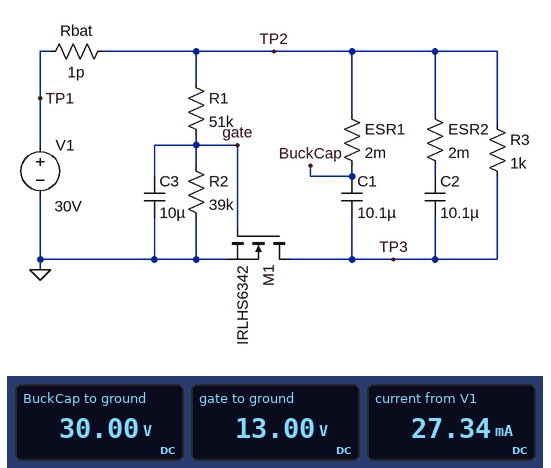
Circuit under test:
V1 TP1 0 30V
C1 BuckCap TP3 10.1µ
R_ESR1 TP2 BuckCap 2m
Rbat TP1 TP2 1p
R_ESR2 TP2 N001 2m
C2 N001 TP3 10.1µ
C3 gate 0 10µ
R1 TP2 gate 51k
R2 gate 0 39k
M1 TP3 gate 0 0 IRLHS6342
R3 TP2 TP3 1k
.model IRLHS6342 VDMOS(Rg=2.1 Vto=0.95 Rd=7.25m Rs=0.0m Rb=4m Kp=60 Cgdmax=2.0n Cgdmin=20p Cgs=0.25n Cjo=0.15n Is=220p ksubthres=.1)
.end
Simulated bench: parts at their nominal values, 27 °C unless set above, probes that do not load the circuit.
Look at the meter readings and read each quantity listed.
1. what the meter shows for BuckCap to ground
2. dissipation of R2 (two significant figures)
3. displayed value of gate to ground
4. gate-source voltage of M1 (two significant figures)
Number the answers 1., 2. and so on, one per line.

1. 30.00 V
2. 4.3 mW
3. 13.00 V
4. 13 V
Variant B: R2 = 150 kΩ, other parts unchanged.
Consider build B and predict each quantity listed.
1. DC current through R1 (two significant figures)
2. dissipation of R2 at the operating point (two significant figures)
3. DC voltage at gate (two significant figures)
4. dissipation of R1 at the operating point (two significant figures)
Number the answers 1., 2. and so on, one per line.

1. 150 µA
2. 3.3 mW
3. 22 V
4. 1.1 mW
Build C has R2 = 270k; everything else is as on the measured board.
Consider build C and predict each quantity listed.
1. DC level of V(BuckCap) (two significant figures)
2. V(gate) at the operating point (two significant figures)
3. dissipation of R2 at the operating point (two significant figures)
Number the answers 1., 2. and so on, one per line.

1. 30 V
2. 25 V
3. 2.4 mW
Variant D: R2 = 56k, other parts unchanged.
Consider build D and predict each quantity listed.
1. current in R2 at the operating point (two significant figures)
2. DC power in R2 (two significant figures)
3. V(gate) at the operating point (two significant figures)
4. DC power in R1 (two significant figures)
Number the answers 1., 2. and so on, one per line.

1. 280 µA
2. 4.4 mW
3. 16 V
4. 4.0 mW
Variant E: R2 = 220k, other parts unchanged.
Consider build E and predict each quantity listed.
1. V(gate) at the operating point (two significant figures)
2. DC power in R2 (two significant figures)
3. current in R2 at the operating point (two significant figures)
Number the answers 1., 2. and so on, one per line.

1. 24 V
2. 2.7 mW
3. 110 µA
